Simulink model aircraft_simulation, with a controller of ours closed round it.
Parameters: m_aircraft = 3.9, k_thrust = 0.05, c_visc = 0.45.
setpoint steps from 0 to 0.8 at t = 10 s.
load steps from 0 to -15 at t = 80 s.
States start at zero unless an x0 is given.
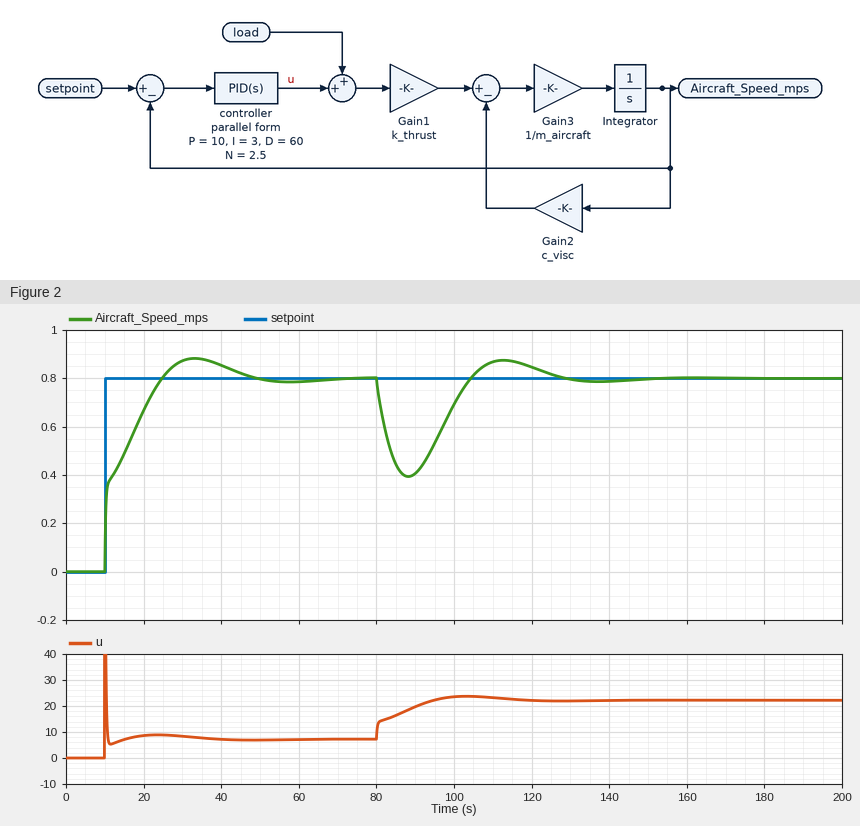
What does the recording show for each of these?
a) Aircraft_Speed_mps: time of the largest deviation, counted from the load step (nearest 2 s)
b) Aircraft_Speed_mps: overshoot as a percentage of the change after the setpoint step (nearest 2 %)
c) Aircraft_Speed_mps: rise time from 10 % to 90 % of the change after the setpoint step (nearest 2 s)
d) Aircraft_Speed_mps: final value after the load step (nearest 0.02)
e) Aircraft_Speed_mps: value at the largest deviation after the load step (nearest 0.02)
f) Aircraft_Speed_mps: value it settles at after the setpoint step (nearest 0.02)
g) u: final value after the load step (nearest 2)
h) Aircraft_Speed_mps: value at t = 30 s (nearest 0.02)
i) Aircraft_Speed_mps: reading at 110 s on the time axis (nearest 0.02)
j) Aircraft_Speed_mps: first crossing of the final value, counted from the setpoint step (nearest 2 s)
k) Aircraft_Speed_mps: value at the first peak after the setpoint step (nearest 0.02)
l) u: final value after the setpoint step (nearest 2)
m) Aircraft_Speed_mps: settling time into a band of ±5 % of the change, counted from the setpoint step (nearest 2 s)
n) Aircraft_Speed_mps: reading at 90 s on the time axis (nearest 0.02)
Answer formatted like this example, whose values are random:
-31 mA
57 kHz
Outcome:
8 s
10 %
12 s
0.80
0.40
0.80
22
0.88
0.86
14 s
0.88
8
32 s
0.40
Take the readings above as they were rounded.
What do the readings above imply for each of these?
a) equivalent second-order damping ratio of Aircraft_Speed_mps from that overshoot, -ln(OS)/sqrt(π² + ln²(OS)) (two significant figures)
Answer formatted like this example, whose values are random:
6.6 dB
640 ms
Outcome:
0.59
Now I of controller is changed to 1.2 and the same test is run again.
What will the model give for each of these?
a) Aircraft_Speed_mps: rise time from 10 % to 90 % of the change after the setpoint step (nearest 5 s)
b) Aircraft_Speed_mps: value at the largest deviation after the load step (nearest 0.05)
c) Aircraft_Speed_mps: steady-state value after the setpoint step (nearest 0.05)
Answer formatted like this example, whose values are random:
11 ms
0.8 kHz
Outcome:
25 s
0.30
0.80
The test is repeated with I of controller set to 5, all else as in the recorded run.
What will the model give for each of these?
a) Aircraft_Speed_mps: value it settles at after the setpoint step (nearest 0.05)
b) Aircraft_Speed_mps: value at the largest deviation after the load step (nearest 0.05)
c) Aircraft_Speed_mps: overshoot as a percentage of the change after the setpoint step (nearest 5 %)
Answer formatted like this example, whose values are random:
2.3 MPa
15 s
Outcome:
0.80
0.45
15 %
